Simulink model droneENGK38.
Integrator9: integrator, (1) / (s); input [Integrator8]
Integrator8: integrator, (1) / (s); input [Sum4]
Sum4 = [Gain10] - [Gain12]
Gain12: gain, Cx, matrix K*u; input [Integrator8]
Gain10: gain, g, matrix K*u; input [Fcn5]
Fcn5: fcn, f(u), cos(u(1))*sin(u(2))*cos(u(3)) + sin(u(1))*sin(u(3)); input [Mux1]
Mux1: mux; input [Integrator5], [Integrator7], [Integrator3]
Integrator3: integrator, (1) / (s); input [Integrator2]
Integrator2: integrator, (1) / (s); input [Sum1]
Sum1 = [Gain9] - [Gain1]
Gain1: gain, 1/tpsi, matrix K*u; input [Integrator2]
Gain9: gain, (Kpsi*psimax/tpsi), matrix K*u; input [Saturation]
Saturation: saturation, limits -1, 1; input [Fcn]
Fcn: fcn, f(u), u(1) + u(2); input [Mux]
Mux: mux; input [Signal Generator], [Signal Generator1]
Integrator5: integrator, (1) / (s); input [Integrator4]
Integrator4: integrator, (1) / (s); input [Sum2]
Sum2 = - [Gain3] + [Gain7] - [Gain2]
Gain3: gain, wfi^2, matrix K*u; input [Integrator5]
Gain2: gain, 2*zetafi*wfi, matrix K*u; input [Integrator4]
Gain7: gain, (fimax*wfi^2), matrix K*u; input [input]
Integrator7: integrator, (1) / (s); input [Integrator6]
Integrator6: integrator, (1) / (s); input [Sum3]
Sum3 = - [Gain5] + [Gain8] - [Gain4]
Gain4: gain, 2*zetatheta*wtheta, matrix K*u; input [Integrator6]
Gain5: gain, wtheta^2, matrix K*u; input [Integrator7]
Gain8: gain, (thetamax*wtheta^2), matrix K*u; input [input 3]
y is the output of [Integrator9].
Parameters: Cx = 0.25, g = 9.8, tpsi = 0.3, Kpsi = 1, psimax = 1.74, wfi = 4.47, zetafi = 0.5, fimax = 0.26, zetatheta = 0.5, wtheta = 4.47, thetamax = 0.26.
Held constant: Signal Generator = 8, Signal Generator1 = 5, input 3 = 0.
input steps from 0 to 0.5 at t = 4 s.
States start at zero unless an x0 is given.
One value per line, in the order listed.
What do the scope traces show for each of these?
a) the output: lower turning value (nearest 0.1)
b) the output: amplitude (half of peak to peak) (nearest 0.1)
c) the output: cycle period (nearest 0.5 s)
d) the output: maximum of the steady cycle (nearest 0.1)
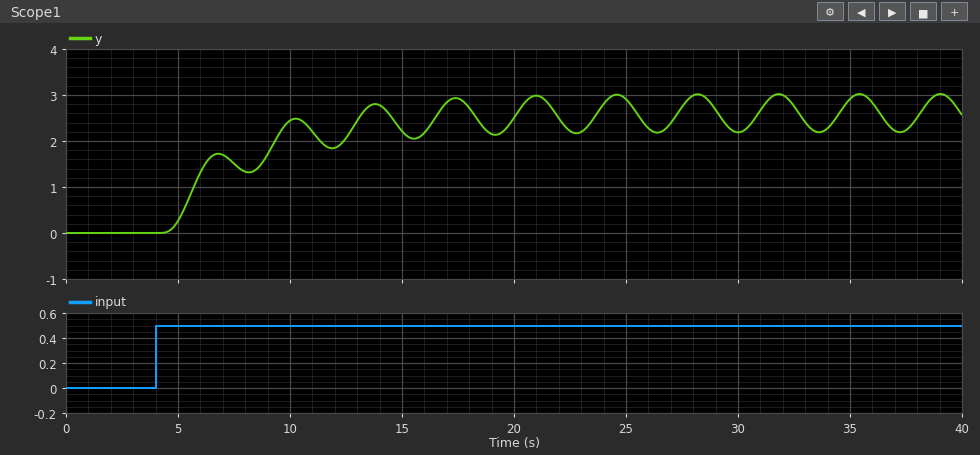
2.2
0.4
3.5 s
3.0
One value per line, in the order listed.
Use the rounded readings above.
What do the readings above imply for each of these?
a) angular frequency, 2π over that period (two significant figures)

1.8 rad/s
